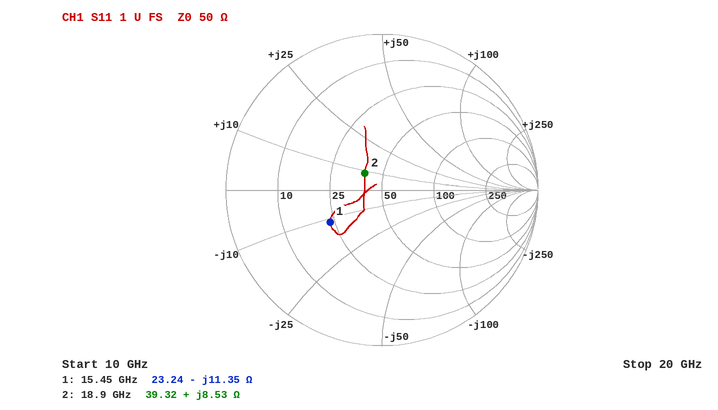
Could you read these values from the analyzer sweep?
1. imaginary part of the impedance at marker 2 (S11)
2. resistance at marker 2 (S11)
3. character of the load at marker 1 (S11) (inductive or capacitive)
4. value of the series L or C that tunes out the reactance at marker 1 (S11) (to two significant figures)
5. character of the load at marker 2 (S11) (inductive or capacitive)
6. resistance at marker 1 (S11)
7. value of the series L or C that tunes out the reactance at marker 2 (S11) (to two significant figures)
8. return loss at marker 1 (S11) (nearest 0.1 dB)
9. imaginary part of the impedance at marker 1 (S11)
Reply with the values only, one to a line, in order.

+8.53 Ω
39.32 Ω
capacitive
120 pH
inductive
23.24 Ω
990 fF
8.1 dB
-11.35 Ω
